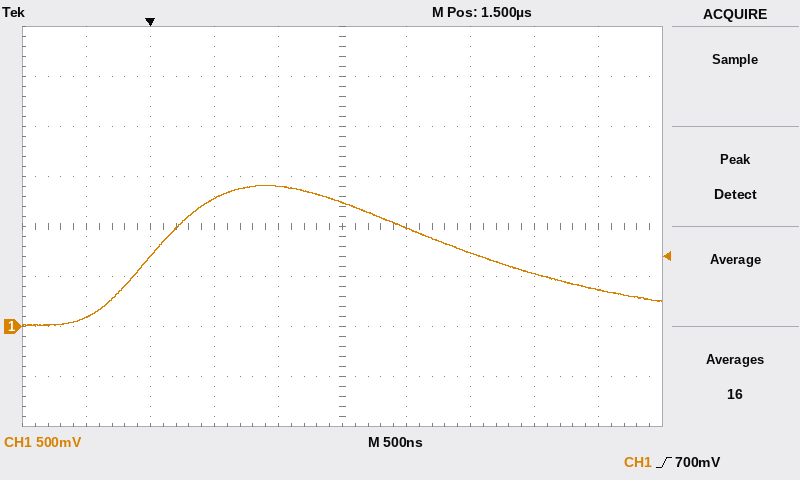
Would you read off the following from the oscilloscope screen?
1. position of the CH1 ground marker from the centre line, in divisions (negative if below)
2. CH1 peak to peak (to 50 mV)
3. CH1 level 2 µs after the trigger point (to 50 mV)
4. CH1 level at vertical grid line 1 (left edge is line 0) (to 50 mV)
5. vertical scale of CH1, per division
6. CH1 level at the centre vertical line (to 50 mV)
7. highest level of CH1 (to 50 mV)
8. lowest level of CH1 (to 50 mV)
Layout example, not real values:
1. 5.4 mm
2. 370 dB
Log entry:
1. -2.0 div
2. 1.40 V
3. 1.00 V
4. 100 mV
5. 500 mV
6. 1.25 V
7. 1.40 V
8. 0 mV
